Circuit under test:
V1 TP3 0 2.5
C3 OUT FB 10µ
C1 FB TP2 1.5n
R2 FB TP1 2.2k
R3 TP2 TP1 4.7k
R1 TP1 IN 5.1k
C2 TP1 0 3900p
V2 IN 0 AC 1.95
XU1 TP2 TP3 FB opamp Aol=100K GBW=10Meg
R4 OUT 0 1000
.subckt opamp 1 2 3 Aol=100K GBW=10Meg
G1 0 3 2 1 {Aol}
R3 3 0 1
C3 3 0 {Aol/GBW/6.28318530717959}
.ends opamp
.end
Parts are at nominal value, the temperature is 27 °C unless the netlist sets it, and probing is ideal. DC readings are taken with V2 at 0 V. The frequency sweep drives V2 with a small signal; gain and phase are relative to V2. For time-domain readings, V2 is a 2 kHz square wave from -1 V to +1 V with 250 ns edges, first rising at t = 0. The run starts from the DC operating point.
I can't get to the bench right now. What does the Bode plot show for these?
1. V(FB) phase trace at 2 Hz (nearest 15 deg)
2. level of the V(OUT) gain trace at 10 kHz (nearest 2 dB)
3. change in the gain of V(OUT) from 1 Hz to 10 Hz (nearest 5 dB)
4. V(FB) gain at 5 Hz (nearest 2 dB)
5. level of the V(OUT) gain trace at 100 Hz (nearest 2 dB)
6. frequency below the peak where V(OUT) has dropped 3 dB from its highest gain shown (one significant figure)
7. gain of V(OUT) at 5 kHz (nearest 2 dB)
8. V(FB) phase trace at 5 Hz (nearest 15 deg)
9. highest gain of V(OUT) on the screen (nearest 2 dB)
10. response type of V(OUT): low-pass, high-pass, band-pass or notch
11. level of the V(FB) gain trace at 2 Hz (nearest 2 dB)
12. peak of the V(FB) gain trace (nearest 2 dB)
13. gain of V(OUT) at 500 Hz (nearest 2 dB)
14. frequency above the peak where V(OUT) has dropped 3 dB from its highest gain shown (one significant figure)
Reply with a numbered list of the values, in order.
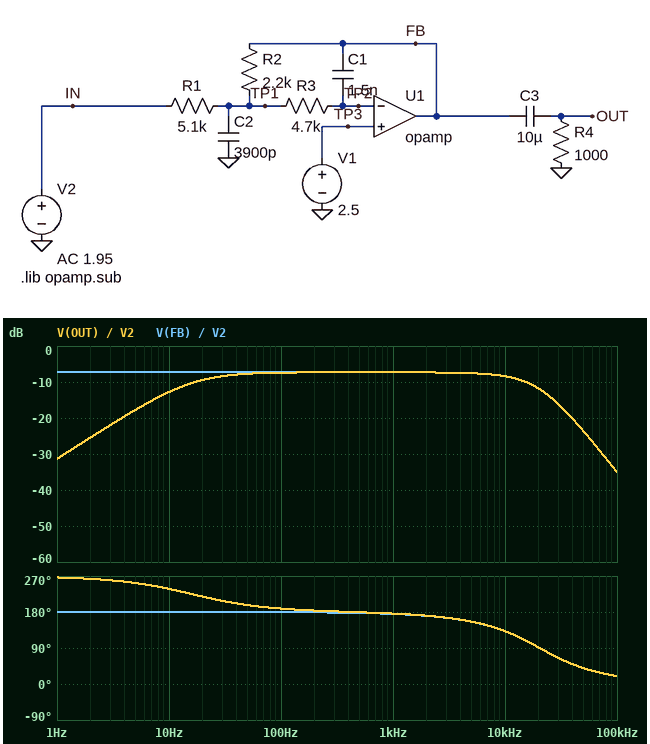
1. 180 deg
2. -8 dB
3. 20 dB
4. -8 dB
5. -8 dB
6. 20 Hz
7. -8 dB
8. 180 deg
9. -8 dB
10. band-pass
11. -8 dB
12. -8 dB
13. -8 dB
14. 20 kHz
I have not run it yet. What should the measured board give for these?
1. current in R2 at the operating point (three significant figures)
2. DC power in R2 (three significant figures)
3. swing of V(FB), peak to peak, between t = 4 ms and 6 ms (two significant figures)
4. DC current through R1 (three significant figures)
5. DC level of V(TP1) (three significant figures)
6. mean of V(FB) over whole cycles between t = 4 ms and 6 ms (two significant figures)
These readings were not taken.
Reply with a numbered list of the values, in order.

1. 490 µA
2. 529 µW
3. 870 mV
4. 490 µA
5. 2.50 V
6. 3.6 V
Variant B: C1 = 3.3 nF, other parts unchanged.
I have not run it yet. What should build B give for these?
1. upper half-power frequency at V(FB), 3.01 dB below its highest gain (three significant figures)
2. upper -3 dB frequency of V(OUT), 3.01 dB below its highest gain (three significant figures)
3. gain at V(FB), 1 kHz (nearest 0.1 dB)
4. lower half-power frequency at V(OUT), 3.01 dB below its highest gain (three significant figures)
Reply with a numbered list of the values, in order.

1. 6.34 kHz
2. 6.37 kHz
3. -7.4 dB
4. 15.8 Hz
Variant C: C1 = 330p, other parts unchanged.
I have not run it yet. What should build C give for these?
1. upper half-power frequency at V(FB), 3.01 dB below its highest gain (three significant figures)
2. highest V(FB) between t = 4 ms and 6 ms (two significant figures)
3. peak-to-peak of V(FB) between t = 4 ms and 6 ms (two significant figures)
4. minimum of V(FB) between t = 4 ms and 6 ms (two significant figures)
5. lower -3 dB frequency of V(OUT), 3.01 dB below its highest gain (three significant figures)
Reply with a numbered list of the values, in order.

1. 51.6 kHz
2. 4.2 V
3. 1.3 V
4. 2.9 V
5. 54.0 Hz
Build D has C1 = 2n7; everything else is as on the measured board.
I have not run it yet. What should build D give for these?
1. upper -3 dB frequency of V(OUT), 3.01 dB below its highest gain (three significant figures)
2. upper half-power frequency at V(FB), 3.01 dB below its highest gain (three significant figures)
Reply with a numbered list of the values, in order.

1. 8.05 kHz
2. 8.02 kHz
